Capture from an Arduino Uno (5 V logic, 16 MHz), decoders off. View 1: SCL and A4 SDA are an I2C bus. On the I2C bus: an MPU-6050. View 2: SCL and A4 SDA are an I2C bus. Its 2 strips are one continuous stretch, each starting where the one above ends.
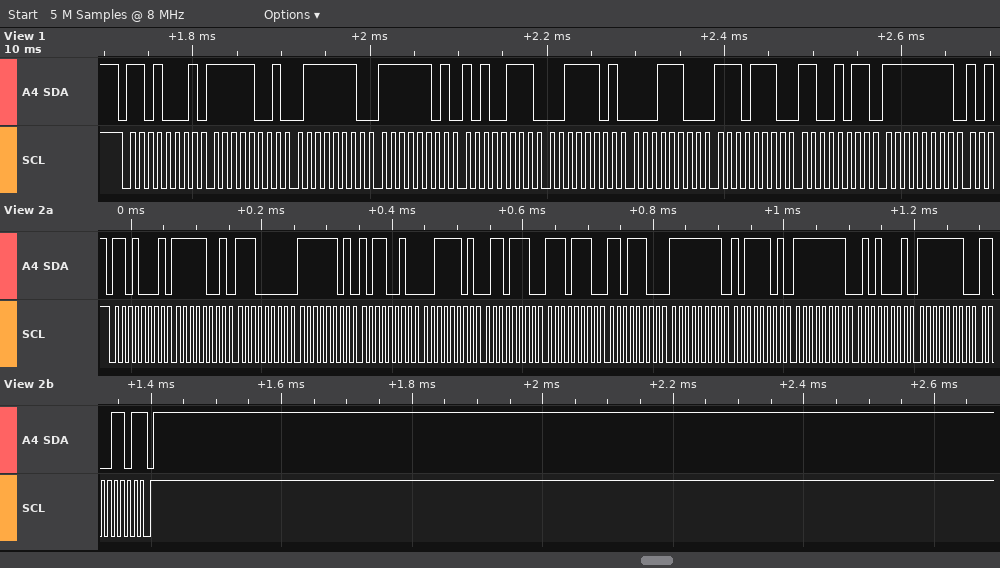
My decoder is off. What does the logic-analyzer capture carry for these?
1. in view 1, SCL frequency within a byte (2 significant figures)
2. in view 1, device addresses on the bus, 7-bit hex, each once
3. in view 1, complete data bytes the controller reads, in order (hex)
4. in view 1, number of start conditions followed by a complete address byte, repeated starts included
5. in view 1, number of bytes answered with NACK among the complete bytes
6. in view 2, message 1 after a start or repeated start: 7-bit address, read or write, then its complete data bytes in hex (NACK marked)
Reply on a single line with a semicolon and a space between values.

100 kHz; 0x68; F9 7E FD A7 3D 1C EE CB FF; 1; 0; 0x68 read: F9 E0 FD B2 3D 6E EE DC FF BD FF 51 FE CD NACK
